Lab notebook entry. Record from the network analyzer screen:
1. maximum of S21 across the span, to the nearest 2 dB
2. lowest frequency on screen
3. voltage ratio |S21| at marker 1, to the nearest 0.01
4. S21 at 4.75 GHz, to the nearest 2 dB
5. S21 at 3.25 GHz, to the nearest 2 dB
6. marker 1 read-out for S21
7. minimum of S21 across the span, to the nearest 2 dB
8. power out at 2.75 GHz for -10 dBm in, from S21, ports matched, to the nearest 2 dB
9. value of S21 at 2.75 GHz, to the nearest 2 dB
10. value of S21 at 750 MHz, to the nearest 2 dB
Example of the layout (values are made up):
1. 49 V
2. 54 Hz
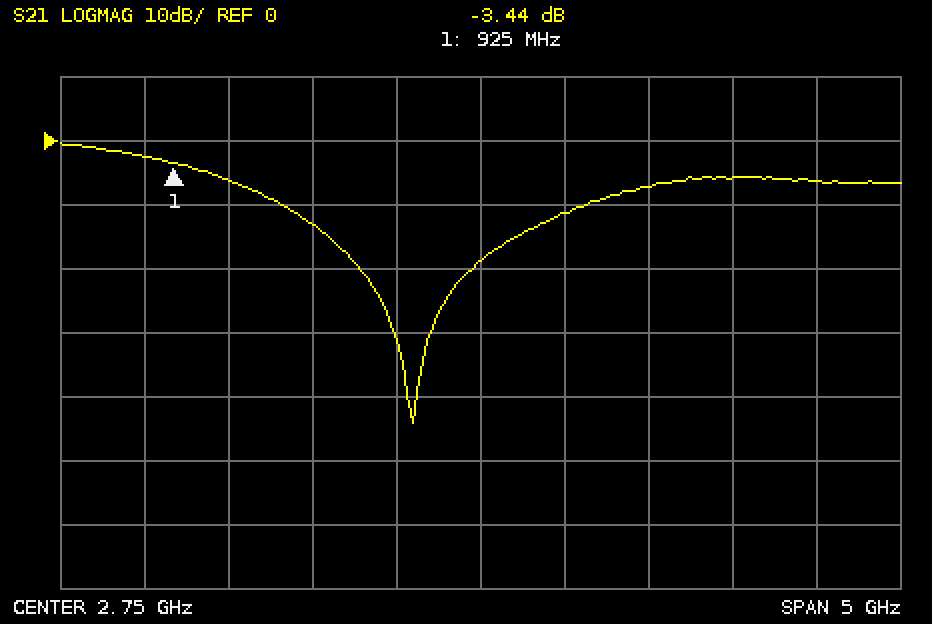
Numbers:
1. 0 dB
2. 250 MHz
3. 0.67
4. -6 dB
5. -12 dB
6. -3.44 dB
7. -44 dB
8. -28 dBm
9. -18 dB
10. -2 dB
